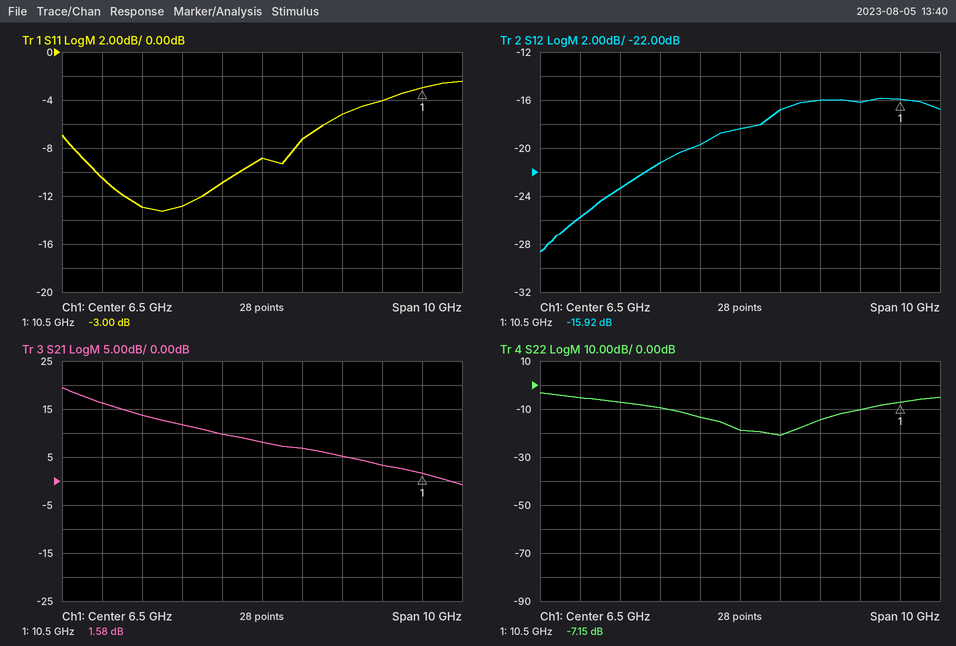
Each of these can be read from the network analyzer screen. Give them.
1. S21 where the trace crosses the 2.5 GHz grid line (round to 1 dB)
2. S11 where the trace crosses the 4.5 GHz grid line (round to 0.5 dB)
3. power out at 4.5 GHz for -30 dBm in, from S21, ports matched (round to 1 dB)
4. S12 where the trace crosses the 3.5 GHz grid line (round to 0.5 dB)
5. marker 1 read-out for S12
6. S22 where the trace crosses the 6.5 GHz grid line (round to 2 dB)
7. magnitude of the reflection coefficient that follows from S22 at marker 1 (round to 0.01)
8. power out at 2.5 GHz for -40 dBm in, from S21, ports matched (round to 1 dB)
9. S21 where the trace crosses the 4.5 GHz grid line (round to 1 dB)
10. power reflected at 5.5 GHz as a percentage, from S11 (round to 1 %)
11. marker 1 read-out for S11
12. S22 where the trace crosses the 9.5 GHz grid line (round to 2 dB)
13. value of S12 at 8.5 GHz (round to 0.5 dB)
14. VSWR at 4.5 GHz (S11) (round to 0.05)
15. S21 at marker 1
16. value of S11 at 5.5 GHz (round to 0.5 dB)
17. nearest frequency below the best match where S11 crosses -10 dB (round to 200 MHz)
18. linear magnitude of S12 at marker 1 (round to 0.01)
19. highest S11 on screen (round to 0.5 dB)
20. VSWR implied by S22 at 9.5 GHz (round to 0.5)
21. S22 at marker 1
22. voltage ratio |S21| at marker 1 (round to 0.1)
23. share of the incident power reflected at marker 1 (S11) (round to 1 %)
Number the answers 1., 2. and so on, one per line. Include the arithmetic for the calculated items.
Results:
1. 16 dB
2. -13.0 dB
3. -30 dBm + (12 dB) = -18 dBm
4. -23.5 dB
5. -15.92 dB
6. -18 dB
7. 10^(-7.15/20) ≈ 0.44
8. -40 dBm + (16 dB) = -24 dBm
9. 12 dB
10. 10^(-11/10) ≈ 8 %
11. -3.00 dB
12. -10 dB
13. -16.0 dB
14. |Γ| = 10^(-13/20) = 0.2239; VSWR = (1 + 0.2239)/(1 − 0.2239) ≈ 1.58, so 1.60 to the nearest 0.05
15. 1.58 dB
16. -11.0 dB
17. 2.4 GHz
18. 10^(-15.92/20) ≈ 0.16
19. -2.5 dB
20. |Γ| = 10^(-10/20) = 0.3162; VSWR = (1 + 0.3162)/(1 − 0.3162) ≈ 1.92, so 2.0 to the nearest 0.5
21. -7.15 dB
22. 10^(1.58/20) ≈ 1.2
23. 10^(-3/10) ≈ 50 %
